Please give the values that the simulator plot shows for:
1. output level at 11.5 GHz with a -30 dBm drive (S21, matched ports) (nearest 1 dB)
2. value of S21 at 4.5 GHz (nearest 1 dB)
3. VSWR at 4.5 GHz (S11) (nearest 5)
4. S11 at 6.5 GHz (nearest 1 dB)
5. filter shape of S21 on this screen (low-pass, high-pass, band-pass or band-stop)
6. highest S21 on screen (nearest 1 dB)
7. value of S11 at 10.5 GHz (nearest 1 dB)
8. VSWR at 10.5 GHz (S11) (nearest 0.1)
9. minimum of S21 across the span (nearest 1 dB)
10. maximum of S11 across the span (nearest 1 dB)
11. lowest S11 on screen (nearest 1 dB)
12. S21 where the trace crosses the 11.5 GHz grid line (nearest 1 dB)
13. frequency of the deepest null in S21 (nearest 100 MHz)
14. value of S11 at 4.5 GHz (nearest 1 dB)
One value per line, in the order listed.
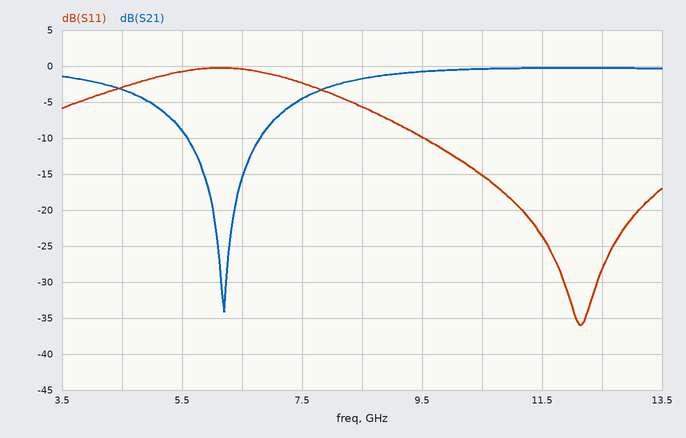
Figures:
-30 dBm
-3 dB
5
0 dB
band-stop
0 dB
-15 dB
1.4
-34 dB
0 dB
-36 dB
0 dB
6.2 GHz
-3 dB
